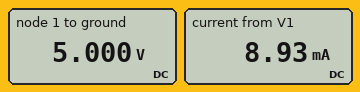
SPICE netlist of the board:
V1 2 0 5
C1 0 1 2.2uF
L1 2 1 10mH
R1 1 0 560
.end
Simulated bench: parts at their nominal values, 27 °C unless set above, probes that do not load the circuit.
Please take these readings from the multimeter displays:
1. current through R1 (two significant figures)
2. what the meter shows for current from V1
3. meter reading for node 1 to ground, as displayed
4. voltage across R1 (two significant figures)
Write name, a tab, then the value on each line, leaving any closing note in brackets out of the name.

current through R1	8.9 mA
what the meter shows for current from V1	8.93 mA
meter reading for node 1 to ground, as displayed	5.000 V
voltage across R1	5.0 V
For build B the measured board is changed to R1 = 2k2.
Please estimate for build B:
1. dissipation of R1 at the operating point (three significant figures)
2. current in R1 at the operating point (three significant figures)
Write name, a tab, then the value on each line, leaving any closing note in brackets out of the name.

dissipation of R1 at the operating point	11.4 mW
current in R1 at the operating point	2.27 mA
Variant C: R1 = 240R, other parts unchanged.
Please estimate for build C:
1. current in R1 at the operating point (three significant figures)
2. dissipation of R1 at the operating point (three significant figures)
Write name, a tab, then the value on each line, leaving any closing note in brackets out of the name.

current in R1 at the operating point	20.8 mA
dissipation of R1 at the operating point	104 mW
